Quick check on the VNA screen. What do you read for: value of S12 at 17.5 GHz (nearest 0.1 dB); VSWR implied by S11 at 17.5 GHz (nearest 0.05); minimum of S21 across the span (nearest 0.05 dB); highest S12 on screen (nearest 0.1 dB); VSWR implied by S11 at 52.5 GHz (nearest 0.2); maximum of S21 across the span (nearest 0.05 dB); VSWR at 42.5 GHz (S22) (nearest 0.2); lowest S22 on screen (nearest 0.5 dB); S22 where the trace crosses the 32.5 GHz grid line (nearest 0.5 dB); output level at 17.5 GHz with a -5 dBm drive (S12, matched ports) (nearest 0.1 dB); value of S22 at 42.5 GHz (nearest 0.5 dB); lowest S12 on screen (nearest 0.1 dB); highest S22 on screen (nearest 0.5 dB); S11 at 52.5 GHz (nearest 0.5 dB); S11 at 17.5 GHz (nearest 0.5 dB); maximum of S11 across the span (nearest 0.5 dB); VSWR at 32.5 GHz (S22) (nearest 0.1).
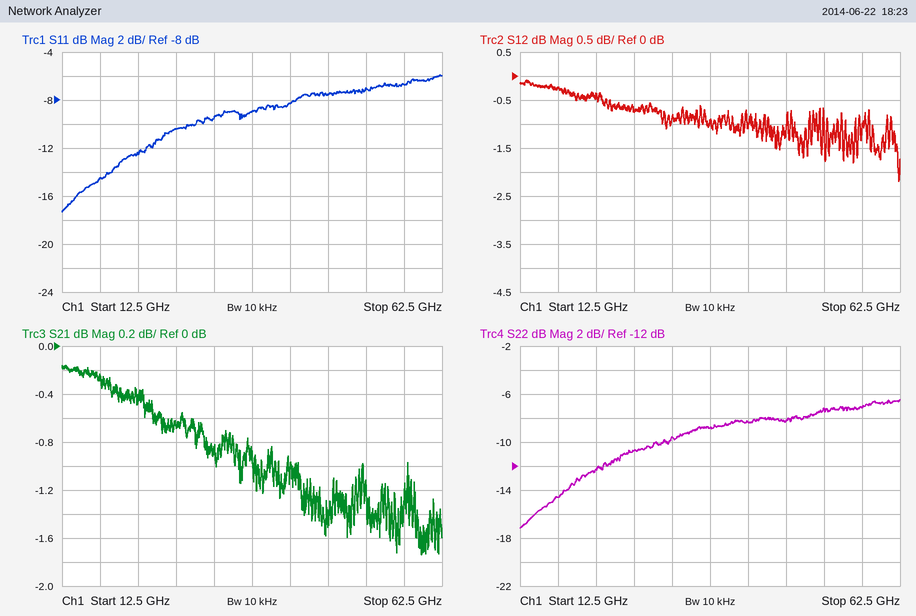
-0.2 dB
1.45
-1.75 dB
-0.1 dB
2.6
-0.15 dB
2.2
-17.0 dB
-9.5 dB
-5.2 dBm
-8.5 dB
-2.2 dB
-6.5 dB
-7.0 dB
-14.5 dB
-6.0 dB
2.0
